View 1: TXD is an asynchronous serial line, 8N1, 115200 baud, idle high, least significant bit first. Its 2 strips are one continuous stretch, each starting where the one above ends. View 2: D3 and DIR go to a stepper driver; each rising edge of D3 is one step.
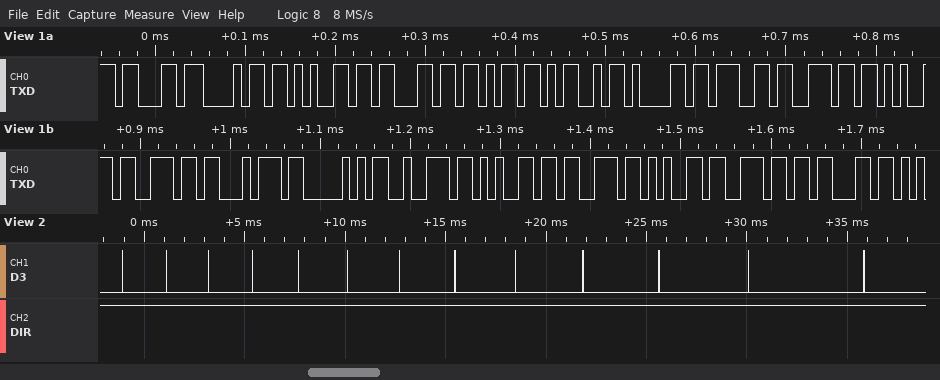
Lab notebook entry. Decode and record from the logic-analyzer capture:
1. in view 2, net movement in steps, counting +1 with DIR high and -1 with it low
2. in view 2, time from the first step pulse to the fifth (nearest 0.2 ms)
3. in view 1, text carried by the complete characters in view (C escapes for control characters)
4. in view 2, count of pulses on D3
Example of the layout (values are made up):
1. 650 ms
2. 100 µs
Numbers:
1. +13
2. 8.8 ms
3. "checkMagnentPresenc"
4. 13
